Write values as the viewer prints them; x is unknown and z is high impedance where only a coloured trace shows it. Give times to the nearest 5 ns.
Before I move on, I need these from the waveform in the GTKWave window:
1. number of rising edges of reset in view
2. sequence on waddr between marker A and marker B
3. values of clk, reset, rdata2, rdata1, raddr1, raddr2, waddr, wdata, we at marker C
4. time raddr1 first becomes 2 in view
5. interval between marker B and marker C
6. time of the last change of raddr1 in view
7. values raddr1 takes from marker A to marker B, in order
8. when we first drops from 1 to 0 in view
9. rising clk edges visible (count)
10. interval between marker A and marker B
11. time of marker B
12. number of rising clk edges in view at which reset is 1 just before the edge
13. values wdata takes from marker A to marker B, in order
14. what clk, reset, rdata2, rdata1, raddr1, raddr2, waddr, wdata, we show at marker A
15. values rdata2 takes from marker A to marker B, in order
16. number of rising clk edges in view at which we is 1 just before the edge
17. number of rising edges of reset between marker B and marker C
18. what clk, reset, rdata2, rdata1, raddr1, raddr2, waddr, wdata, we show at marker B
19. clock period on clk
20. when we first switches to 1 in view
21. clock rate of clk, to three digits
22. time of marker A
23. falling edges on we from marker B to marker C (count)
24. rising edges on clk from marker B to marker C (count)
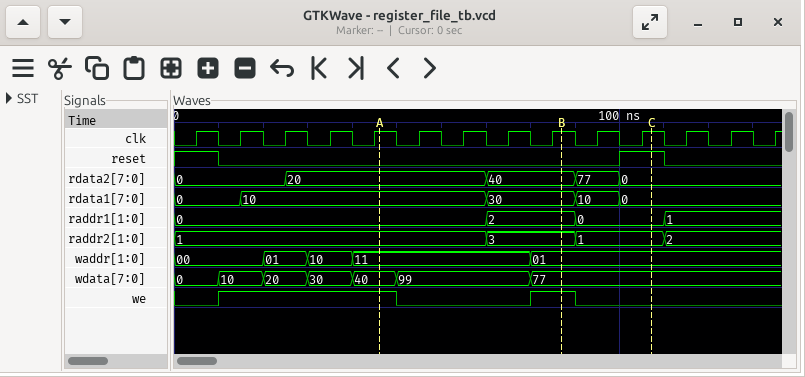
1
11, 01
clk=1, reset=1, rdata2=0, rdata1=0, raddr1=0, raddr2=1, waddr=01, wdata=77, we=0
70 ns
20 ns
110 ns
0, 2
50 ns
14
40 ns
85 ns
2
40, 99, 77
clk=1, reset=0, rdata2=20, rdata1=10, raddr1=0, raddr2=1, waddr=11, wdata=40, we=1
20, 40
5
1
clk=1, reset=0, rdata2=40, rdata1=30, raddr1=2, raddr2=3, waddr=01, wdata=77, we=1
10 ns
10 ns
100 MHz
45 ns
1
2
